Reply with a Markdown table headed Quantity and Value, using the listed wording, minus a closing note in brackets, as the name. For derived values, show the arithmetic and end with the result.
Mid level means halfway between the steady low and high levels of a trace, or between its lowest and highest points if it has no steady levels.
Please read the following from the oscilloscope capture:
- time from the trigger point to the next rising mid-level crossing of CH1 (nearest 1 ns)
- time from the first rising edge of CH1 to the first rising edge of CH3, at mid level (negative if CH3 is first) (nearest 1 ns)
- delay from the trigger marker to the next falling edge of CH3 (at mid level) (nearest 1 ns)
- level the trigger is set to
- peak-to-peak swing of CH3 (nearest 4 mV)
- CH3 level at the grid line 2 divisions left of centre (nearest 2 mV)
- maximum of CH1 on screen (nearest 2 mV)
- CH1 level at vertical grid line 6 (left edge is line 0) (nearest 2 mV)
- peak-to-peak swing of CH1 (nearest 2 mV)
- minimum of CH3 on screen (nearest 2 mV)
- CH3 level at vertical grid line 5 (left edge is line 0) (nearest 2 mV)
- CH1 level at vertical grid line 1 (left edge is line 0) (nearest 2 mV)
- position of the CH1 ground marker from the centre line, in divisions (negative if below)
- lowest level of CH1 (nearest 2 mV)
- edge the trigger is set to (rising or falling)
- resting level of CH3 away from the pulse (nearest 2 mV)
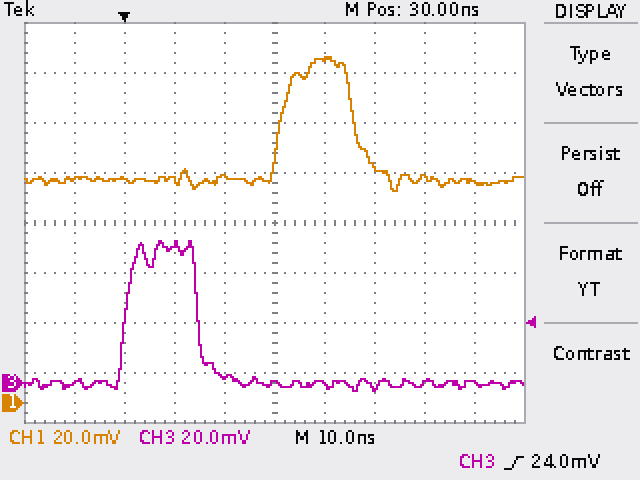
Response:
| Quantity | Value |
|---|---|
| time from the trigger point to the next rising mid-level crossing of CH1 | 31 ns |
| time from the first rising edge of CH1 to the first rising edge of CH3, at mid level (negative if CH3 is first) | -31 ns |
| delay from the trigger marker to the next falling edge of CH3 (at mid level) | 15 ns |
| level the trigger is set to | 24.0 mV |
| peak-to-peak swing of CH3 | 60 mV |
| CH3 level at the grid line 2 divisions left of centre | 56 mV |
| maximum of CH1 on screen | 138 mV |
| CH1 level at vertical grid line 6 (left edge is line 0) | 138 mV |
| peak-to-peak swing of CH1 | 138 mV − (84 mV) = 54 mV |
| minimum of CH3 on screen | -4 mV |
| CH3 level at vertical grid line 5 (left edge is line 0) | 0 mV |
| CH1 level at vertical grid line 1 (left edge is line 0) | 90 mV |
| position of the CH1 ground marker from the centre line, in divisions | -3.6 div |
| lowest level of CH1 | 84 mV |
| edge the trigger is set to | rising |
| resting level of CH3 away from the pulse | 0 mV |
